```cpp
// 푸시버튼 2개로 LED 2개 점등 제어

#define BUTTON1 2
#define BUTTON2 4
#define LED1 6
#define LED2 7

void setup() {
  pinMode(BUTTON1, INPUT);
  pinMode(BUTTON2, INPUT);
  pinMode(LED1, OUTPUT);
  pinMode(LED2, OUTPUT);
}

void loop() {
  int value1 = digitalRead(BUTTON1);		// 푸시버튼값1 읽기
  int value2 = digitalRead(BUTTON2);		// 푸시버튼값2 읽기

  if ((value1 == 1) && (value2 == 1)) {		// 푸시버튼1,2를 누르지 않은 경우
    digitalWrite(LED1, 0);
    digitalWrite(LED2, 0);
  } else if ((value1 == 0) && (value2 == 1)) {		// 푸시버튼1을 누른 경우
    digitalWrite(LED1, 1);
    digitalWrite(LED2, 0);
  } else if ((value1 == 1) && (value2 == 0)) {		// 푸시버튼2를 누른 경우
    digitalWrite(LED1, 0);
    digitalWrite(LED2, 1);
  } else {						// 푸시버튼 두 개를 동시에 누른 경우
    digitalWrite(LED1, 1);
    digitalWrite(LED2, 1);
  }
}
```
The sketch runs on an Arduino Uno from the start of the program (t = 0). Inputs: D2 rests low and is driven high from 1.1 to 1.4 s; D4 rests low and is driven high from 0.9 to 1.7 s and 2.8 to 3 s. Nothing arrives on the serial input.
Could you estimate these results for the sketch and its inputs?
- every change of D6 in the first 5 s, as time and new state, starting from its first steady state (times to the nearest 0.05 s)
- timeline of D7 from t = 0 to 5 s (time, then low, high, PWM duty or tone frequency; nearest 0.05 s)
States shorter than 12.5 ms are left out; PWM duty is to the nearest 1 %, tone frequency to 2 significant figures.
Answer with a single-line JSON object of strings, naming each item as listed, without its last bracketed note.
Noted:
{"every change of D6 in the first 5 s, as time and new state, starting from its first steady state": "0 s high; 1.1 s low; 1.4 s high", "timeline of D7 from t = 0 to 5 s": "0 s high; 0.9 s low; 1.7 s high; 2.8 s low; 3 s high"}
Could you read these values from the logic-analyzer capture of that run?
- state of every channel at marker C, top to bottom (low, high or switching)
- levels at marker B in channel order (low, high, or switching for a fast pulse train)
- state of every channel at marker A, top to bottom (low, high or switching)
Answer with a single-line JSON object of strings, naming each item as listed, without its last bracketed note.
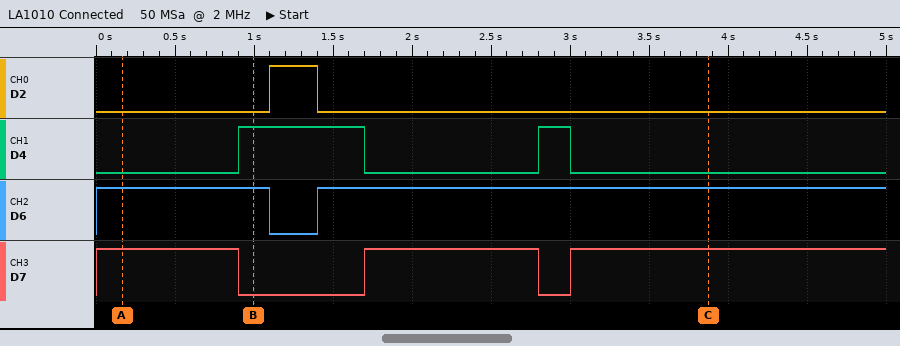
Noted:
{"state of every channel at marker C, top to bottom": "D2 low, D4 low, D6 high, D7 high", "levels at marker B in channel order": "D2 low, D4 high, D6 high, D7 low", "state of every channel at marker A, top to bottom": "D2 low, D4 low, D6 high, D7 high"}
